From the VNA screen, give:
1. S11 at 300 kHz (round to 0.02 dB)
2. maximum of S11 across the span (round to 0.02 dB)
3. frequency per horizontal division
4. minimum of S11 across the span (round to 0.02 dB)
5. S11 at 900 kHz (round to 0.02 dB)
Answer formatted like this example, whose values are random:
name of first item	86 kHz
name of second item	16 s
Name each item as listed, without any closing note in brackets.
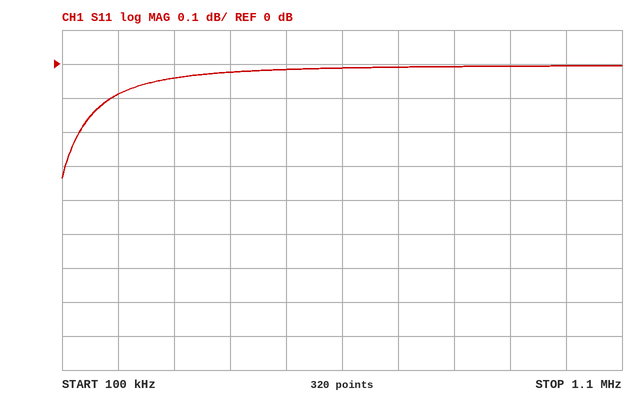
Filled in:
S11 at 300 kHz	-0.04 dB
maximum of S11 across the span	0.00 dB
frequency per horizontal division	100 kHz
minimum of S11 across the span	-0.34 dB
S11 at 900 kHz	0.00 dB
